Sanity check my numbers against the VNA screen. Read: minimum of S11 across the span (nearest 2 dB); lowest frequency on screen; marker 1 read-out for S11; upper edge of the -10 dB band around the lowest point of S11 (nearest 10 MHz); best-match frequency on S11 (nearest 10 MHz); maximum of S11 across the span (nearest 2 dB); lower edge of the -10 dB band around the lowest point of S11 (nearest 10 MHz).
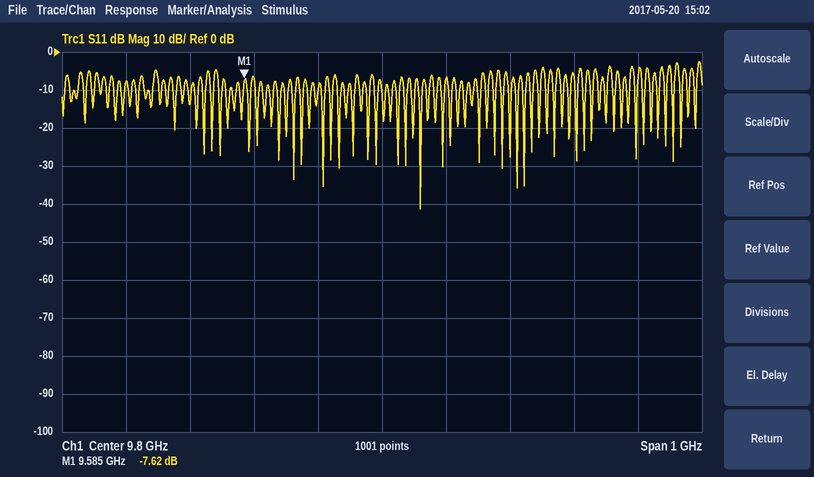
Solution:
-42 dB
9.3 GHz
-7.62 dB
9.86 GHz
9.86 GHz
-2 dB
9.86 GHz
